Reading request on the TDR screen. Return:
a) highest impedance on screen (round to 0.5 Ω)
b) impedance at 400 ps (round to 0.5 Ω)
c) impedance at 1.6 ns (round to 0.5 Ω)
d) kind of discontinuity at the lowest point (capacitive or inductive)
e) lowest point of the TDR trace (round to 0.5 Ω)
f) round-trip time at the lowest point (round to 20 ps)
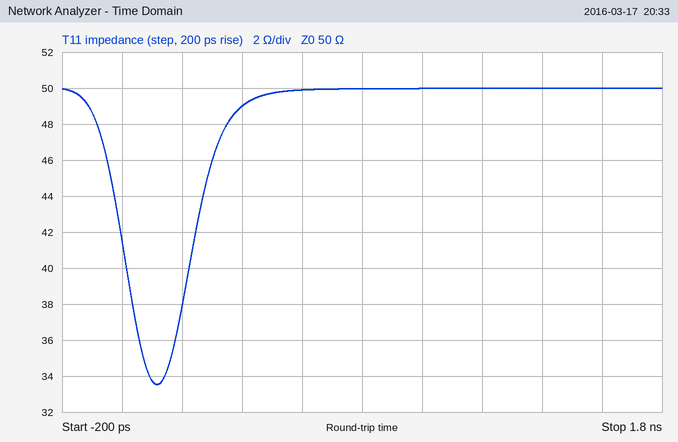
50.0 Ω
49.0 Ω
50.0 Ω
capacitive
33.5 Ω
120 ps
